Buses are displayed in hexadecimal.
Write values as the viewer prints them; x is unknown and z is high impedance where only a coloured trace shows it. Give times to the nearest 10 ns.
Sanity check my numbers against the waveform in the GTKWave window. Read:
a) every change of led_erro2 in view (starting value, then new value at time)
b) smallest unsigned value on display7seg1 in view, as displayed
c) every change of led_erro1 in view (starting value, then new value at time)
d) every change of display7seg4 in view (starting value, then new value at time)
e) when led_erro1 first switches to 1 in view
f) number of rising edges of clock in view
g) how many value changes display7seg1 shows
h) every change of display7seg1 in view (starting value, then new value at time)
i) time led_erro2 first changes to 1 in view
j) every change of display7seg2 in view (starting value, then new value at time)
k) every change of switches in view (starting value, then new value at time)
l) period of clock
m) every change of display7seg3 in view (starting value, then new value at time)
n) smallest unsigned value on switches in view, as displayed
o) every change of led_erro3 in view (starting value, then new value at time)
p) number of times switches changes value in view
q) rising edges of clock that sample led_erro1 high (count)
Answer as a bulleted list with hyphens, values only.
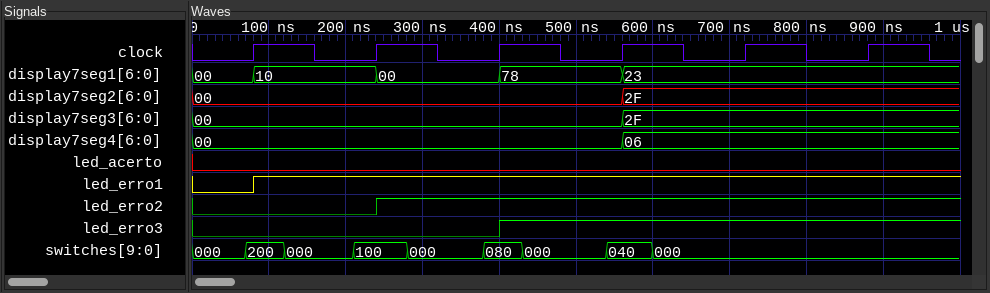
- 0, 1 at 240 ns
- 00
- 0, 1 at 80 ns
- 00, 06 at 560 ns
- 80 ns
- 6
- 4
- 00, 10 at 80 ns, 00 at 240 ns, 78 at 400 ns, 23 at 560 ns
- 240 ns
- 00, 2F at 560 ns
- 000, 200 at 70 ns, 000 at 120 ns, 100 at 210 ns, 000 at 280 ns, 080 at 380 ns, 000 at 430 ns, 040 at 540 ns, 000 at 600 ns
- 160 ns
- 00, 2F at 560 ns
- 000
- 0, 1 at 400 ns
- 8
- 5
